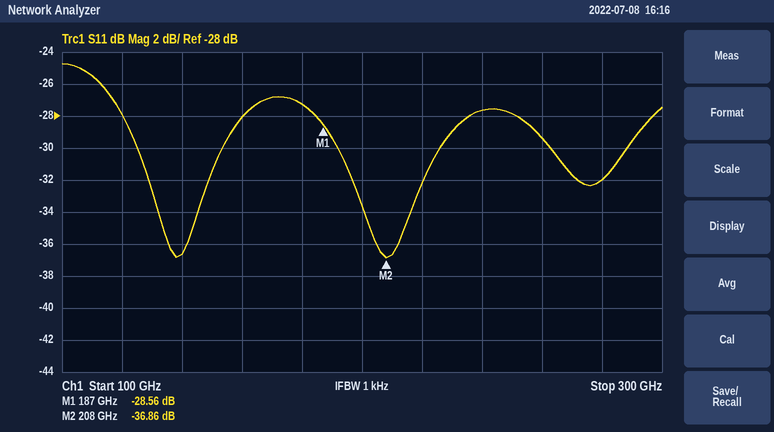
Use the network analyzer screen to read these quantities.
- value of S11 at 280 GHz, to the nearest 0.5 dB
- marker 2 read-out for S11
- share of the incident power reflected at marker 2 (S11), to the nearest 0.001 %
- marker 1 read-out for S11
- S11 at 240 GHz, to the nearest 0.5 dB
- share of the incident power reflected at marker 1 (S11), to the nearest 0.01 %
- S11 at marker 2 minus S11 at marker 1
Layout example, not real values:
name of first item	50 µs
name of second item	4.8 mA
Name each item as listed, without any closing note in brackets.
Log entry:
value of S11 at 280 GHz, to the nearest 0.5 dB	-32.0 dB
marker 2 read-out for S11	-36.86 dB
share of the incident power reflected at marker 2 (S11), to the nearest 0.001 %	0.021 %
marker 1 read-out for S11	-28.56 dB
S11 at 240 GHz, to the nearest 0.5 dB	-27.5 dB
share of the incident power reflected at marker 1 (S11), to the nearest 0.01 %	0.14 %
S11 at marker 2 minus S11 at marker 1	-8.30 dB
